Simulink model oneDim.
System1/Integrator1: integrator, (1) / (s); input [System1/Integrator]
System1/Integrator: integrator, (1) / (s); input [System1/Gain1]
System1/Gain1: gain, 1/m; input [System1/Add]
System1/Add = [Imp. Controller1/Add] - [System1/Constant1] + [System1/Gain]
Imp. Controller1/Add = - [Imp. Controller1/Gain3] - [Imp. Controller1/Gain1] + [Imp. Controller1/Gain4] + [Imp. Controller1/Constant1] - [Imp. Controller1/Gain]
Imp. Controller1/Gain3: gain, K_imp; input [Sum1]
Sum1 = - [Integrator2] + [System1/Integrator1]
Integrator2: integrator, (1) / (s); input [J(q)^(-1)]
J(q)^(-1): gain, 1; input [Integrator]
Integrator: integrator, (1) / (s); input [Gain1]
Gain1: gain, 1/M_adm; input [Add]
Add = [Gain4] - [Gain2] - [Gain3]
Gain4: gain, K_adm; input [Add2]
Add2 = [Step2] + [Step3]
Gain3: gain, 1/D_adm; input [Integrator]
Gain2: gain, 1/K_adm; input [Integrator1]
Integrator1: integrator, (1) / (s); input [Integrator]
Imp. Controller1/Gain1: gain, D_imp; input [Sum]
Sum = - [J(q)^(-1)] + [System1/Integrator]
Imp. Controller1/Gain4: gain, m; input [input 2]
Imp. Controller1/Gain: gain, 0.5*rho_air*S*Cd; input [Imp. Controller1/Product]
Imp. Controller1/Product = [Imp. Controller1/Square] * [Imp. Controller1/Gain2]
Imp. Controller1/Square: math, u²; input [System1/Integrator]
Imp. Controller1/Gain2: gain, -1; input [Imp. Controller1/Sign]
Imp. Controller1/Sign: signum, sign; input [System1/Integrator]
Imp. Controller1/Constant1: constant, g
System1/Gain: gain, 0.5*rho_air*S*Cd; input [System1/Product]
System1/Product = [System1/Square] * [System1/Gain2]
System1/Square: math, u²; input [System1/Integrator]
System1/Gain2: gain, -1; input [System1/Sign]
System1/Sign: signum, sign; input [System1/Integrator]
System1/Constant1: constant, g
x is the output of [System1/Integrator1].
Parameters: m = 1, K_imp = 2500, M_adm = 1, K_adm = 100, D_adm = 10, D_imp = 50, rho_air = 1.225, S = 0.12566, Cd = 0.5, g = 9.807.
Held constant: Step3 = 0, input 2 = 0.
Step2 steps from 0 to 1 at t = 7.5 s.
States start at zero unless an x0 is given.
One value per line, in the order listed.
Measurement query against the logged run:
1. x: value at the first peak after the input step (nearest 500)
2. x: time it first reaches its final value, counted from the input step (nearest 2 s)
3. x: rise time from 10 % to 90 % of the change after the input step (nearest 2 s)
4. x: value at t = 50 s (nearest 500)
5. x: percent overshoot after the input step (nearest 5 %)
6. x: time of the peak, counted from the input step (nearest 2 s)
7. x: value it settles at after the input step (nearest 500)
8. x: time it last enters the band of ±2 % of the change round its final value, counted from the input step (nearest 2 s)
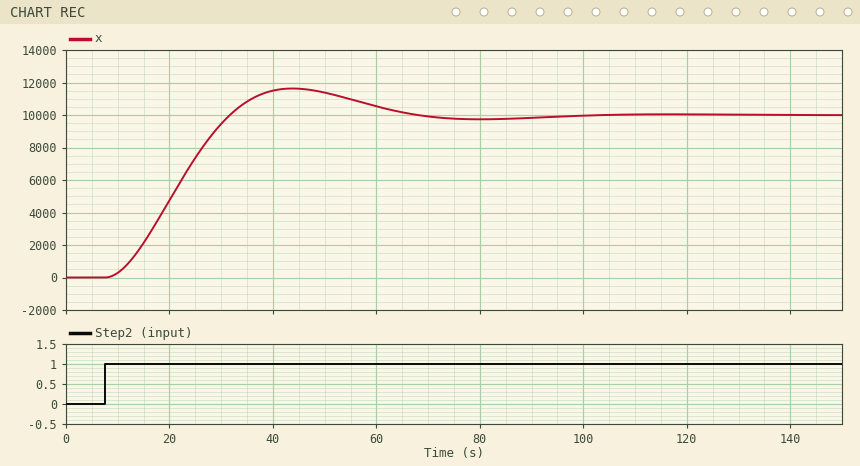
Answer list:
11500
24 s
16 s
11500
15 %
36 s
10000
80 s
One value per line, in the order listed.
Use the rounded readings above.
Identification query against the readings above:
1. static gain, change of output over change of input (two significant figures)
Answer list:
10000
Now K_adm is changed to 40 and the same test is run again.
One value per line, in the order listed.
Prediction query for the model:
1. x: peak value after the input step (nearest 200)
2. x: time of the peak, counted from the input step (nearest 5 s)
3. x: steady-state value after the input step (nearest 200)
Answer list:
2200
20 s
1600
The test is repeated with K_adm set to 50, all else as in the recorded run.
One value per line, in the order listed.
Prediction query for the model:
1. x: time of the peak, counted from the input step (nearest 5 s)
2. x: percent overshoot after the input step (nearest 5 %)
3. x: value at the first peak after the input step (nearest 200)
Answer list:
25 s
30 %
3200
